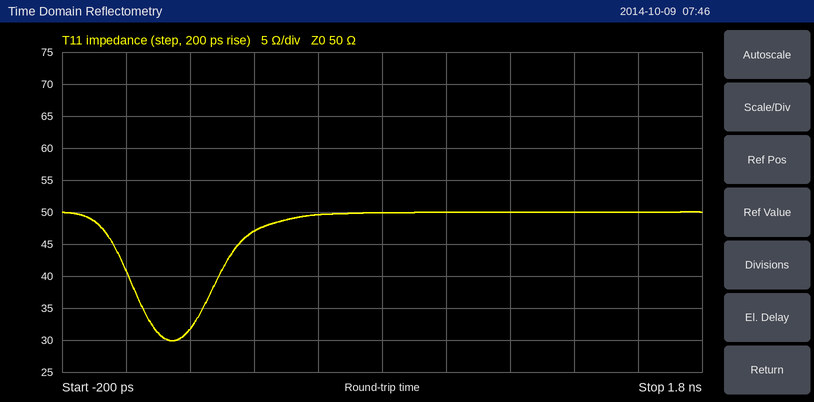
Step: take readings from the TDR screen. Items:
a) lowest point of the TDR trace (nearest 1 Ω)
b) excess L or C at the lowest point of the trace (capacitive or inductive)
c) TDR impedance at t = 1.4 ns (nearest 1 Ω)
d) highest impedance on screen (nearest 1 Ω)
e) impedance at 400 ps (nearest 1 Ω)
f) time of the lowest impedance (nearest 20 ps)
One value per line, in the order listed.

30 Ω
capacitive
50 Ω
50 Ω
47 Ω
140 ps
